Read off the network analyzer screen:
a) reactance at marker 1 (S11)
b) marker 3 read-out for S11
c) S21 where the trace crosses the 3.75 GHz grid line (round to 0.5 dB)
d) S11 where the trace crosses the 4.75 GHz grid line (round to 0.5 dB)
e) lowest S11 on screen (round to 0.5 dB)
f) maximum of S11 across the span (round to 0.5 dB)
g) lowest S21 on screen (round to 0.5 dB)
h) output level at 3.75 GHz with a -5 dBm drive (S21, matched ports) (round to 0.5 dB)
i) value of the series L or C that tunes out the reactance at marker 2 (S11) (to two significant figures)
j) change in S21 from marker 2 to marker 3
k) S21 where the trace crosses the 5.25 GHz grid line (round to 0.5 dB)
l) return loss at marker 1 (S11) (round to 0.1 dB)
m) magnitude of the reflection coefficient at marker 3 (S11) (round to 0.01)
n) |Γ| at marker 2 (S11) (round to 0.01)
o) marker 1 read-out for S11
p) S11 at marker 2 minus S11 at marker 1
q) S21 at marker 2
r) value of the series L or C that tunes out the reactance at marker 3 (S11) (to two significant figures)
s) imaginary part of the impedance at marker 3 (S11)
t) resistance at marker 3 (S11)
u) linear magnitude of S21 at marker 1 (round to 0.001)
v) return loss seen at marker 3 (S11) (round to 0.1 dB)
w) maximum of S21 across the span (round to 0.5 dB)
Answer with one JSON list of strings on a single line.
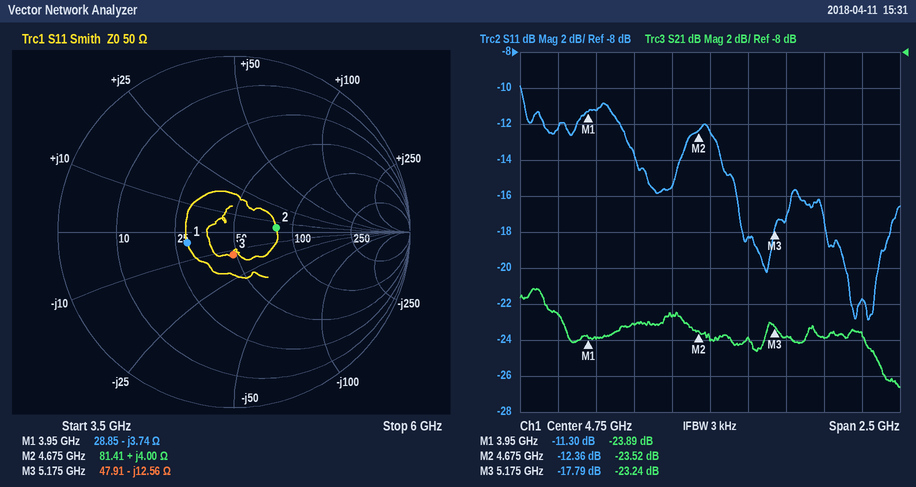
["-3.74 Ω", "-17.79 dB", "-22.5 dB", "-12.5 dB", "-23.0 dB", "-10.0 dB", "-26.5 dB", "-27.5 dBm", "8.5 pF", "0.28 dB", "-24.0 dB", "11.3 dB", "0.13", "0.24", "-11.30 dB", "-1.06 dB", "-23.52 dB", "390 pH", "-12.56 Ω", "47.91 Ω", "0.064", "17.8 dB", "-21.0 dB"]
